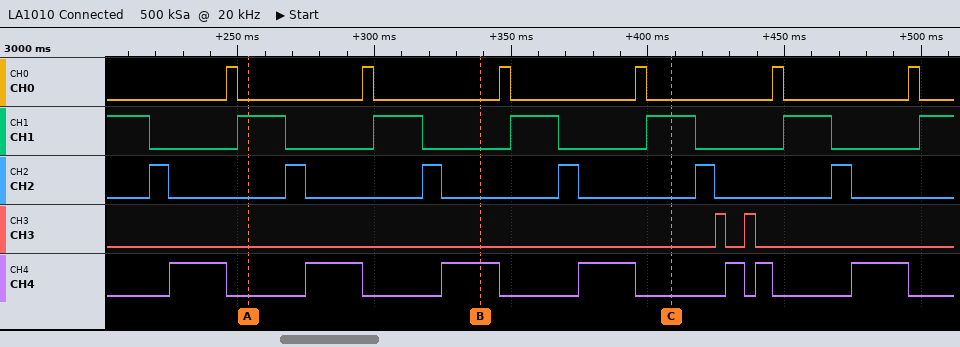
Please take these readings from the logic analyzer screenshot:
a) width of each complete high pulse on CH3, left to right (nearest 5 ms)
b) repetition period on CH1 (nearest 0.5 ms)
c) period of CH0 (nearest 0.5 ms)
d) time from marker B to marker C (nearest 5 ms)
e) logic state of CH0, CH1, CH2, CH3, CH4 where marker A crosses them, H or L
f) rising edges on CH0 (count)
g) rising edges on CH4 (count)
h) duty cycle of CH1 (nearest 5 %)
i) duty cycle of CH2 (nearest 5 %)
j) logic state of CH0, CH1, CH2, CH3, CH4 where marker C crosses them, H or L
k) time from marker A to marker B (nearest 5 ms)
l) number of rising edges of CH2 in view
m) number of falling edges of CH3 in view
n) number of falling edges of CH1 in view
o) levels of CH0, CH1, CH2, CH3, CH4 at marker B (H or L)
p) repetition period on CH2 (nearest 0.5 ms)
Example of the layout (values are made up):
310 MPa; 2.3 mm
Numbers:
5 ms, 5 ms; 50 ms; 50 ms; 70 ms; CH0=L, CH1=H, CH2=L, CH3=L, CH4=L; 6; 7; 35 %; 15 %; CH0=L, CH1=H, CH2=L, CH3=L, CH4=L; 85 ms; 6; 2; 6; CH0=L, CH1=L, CH2=L, CH3=L, CH4=H; 50 ms
